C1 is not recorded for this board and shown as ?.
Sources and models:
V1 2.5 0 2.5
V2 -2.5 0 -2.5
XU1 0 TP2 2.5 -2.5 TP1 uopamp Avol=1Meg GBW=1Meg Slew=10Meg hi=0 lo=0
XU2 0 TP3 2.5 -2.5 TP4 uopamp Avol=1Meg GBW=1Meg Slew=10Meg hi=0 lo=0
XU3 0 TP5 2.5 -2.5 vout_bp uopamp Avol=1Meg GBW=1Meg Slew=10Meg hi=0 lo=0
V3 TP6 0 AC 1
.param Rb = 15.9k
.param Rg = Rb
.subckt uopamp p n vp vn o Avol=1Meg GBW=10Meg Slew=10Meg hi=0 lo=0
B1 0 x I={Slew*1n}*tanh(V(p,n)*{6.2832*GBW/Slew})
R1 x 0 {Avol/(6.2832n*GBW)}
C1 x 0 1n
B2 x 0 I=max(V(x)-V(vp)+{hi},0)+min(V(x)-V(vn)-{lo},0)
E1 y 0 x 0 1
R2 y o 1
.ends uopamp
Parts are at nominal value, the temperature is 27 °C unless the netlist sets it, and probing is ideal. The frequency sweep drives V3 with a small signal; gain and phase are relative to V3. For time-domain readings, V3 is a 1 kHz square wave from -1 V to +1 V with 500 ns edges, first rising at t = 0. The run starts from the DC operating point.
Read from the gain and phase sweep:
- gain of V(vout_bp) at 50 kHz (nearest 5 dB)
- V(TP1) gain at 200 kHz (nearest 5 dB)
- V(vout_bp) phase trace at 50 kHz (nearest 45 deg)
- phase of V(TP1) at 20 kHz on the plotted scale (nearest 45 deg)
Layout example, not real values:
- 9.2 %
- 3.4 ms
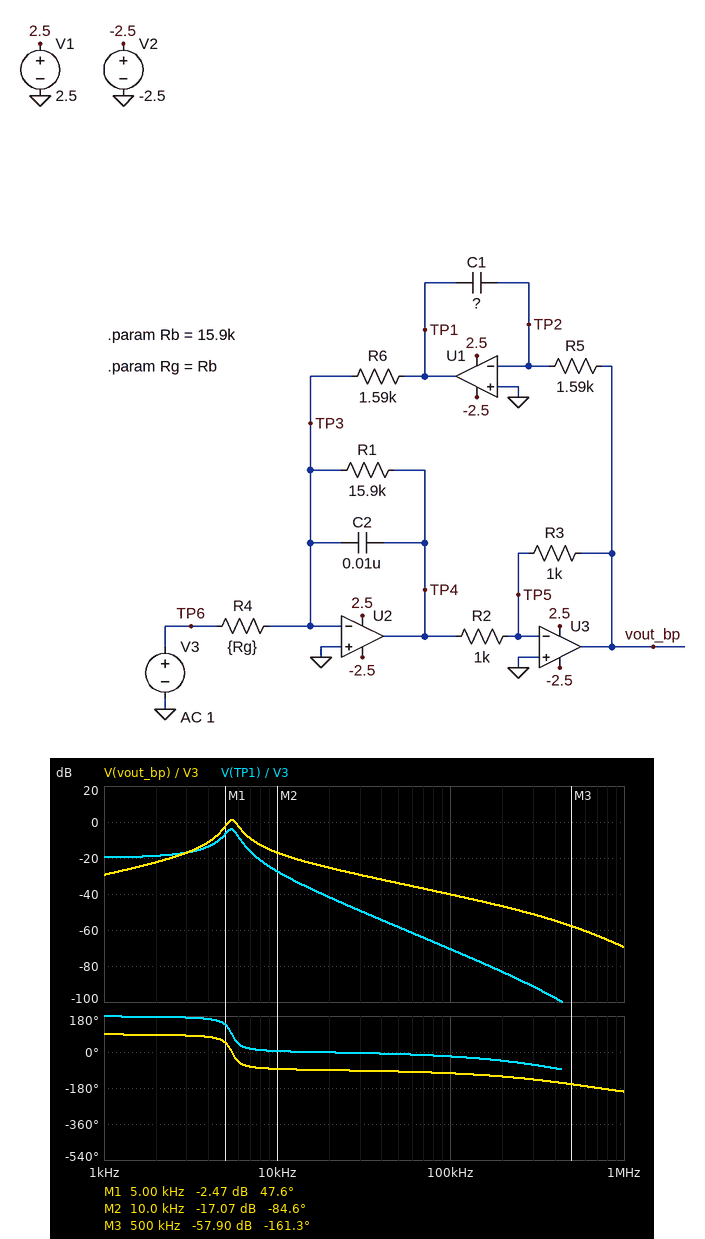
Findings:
- -35 dB
- -85 dB
- -90 deg
- 0 deg
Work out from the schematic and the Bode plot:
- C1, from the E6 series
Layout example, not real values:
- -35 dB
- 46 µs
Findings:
- 33 nF
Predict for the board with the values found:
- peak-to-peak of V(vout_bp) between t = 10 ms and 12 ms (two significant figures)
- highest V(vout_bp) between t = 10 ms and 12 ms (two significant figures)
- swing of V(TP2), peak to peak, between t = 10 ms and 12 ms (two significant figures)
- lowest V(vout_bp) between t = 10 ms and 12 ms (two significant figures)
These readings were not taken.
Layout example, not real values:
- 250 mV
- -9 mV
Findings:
- 660 mV
- 330 mV
- 2.0 mV
- -330 mV
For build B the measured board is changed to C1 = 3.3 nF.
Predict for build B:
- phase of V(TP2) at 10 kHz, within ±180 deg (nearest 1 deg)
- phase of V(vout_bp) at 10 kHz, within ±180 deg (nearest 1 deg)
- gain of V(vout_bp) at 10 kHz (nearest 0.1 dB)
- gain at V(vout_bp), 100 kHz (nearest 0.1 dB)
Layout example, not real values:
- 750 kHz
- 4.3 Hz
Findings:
- 88 deg
- 89 deg
- -25.7 dB
- -40.1 dB
